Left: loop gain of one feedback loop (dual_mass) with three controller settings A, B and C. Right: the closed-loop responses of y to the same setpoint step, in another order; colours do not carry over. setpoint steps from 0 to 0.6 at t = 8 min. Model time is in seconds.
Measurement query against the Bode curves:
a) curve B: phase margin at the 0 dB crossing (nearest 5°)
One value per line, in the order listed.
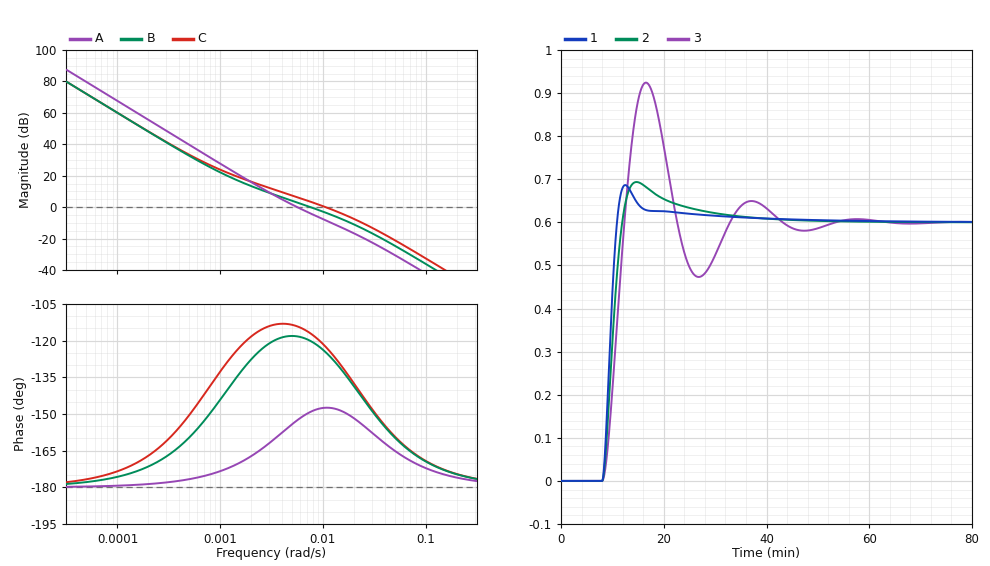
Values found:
60°
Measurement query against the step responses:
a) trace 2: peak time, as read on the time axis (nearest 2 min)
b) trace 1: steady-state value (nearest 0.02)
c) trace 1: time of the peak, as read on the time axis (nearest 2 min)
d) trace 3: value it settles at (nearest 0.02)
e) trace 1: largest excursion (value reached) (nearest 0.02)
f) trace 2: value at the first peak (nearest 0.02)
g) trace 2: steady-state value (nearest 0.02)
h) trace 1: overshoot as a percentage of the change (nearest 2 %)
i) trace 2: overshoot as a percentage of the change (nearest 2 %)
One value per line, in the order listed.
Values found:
14 min
0.60
12 min
0.60
0.68
0.70
0.60
14 %
16 %
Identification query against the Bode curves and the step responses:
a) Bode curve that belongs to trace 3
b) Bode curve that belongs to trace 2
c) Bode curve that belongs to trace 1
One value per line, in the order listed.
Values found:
A
B
C
